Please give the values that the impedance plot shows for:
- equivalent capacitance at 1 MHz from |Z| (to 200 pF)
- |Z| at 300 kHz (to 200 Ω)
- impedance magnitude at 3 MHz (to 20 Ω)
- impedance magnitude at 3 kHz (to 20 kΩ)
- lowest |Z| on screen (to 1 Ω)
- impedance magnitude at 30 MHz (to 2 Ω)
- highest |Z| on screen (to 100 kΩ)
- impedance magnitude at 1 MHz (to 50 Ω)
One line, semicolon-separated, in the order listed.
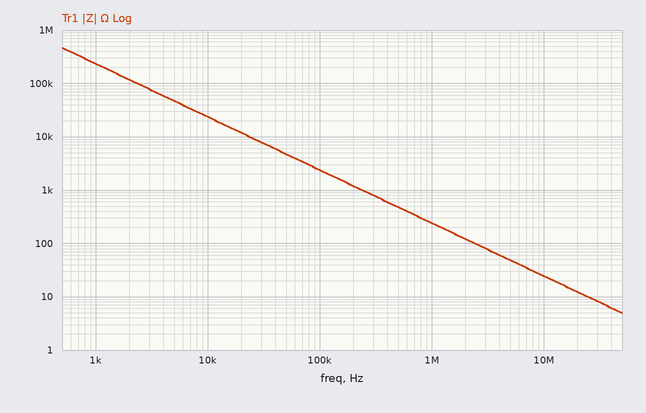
600 pF; 800 Ω; 80 Ω; 80 kΩ; 5 Ω; 8 Ω; 500 kΩ; 250 Ω
